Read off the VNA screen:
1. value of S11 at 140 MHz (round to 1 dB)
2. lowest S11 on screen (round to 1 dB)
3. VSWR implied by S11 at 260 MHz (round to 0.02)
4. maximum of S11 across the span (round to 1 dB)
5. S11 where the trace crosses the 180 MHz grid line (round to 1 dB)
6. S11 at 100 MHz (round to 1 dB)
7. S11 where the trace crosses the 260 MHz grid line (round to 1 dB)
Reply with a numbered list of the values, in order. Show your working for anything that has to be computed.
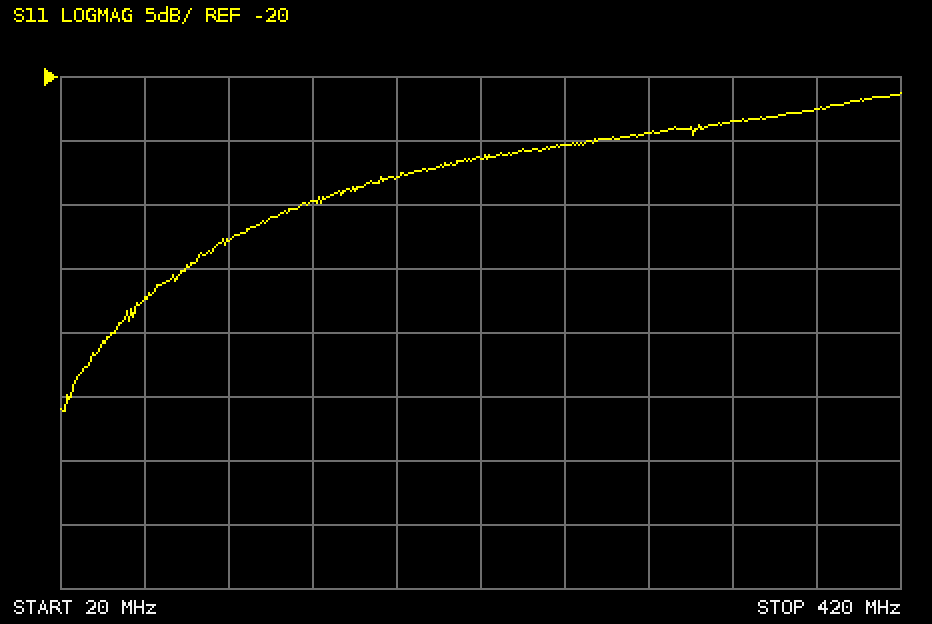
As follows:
1. -30 dB
2. -46 dB
3. |Γ| = 10^(-25/20) = 0.0562; VSWR = (1 + 0.0562)/(1 − 0.0562) ≈ 1.12
4. -21 dB
5. -28 dB
6. -33 dB
7. -25 dB
